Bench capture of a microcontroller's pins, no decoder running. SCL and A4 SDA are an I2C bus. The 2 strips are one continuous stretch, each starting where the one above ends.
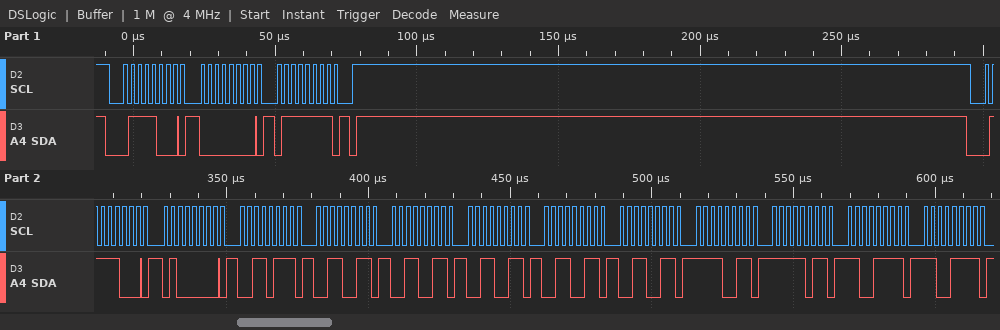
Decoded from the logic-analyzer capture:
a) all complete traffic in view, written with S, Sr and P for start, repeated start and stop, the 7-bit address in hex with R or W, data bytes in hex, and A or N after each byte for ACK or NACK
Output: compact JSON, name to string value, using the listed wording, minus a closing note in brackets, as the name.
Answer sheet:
{"all complete traffic in view, written with S, Sr and P for start, repeated start and stop, the 7-bit address in hex with R or W, data bytes in hex, and A or N after each byte for ACK or NACK": "S 3CW A 00 A 7F A P S 3CW A 40 A 37 A 33 A 33 A 33 A 33 A 33 A F3 A FB A CF A CF A"}
